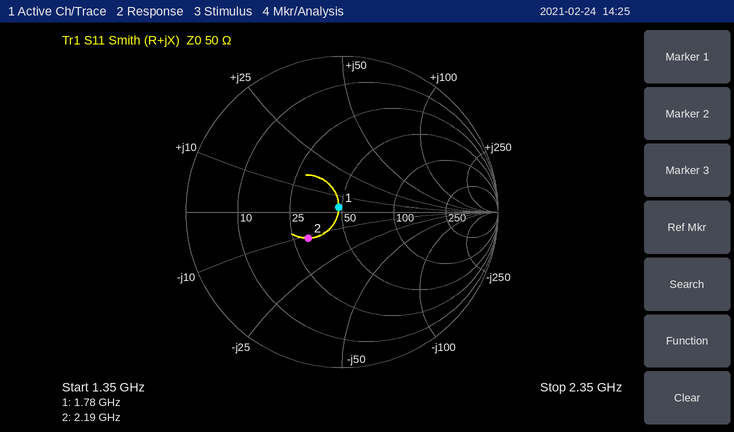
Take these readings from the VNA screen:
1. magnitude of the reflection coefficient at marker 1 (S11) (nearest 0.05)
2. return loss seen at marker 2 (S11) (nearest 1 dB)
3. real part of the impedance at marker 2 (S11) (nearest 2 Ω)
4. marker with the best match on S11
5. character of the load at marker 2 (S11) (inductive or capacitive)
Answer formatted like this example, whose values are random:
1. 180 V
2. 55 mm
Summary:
1. 0.05
2. 11 dB
3. 30 Ω
4. marker 1
5. capacitive
